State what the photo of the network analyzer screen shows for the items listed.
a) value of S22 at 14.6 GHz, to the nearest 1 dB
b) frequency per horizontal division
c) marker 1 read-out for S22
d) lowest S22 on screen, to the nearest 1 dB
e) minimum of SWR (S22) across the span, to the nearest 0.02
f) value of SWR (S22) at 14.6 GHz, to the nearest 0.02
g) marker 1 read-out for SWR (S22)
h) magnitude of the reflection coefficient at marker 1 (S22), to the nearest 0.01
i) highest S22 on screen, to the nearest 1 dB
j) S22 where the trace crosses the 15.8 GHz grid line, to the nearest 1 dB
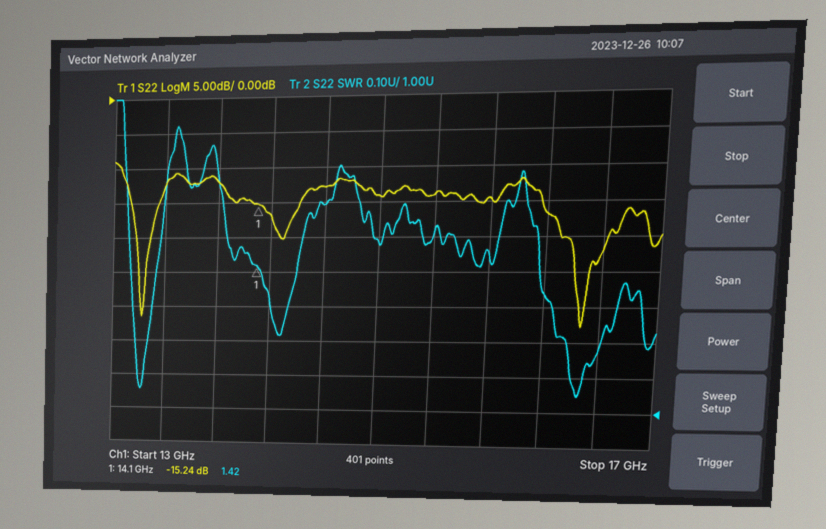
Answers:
-13 dB
400 MHz
-15.24 dB
-33 dB
1.04
1.60
1.42
0.17
-9 dB
-15 dB
